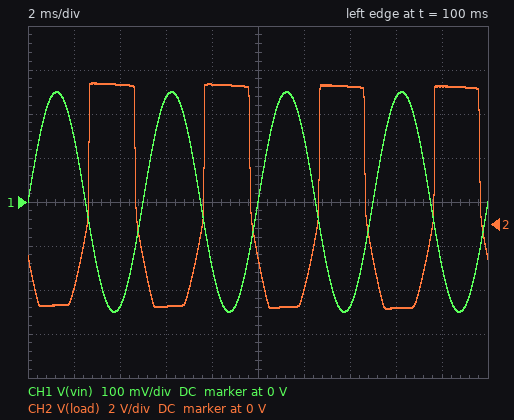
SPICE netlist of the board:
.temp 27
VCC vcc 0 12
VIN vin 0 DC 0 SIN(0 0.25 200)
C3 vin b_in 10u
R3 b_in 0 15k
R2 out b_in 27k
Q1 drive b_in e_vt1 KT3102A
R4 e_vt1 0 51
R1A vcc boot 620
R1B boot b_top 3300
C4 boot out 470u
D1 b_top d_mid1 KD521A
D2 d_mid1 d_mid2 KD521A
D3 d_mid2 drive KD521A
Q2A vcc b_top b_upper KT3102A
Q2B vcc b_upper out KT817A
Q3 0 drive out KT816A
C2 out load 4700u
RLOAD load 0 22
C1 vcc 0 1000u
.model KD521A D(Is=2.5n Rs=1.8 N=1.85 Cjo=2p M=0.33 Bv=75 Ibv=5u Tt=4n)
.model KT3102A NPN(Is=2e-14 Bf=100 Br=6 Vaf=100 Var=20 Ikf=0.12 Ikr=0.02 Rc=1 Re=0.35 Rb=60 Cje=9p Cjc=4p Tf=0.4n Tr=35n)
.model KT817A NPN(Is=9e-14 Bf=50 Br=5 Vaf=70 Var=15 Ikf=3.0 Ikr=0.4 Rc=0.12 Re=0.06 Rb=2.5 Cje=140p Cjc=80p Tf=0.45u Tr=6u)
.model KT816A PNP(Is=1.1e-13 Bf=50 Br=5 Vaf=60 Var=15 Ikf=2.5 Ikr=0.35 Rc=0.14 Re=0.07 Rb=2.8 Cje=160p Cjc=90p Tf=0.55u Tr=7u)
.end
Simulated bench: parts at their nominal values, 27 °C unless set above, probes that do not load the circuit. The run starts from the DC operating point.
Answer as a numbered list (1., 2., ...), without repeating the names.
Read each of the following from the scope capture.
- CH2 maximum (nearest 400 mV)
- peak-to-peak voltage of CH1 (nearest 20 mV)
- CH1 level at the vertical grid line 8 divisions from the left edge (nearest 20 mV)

1. 6.4 V
2. 500 mV
3. 240 mV
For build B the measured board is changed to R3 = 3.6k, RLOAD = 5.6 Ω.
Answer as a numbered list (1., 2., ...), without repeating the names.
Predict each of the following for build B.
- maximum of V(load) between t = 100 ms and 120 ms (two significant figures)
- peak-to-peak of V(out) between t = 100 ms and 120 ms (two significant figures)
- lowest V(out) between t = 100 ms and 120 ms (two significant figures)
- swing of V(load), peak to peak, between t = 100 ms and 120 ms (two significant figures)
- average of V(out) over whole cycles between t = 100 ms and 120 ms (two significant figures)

1. 3.0 V
2. 4.7 V
3. 6.4 V
4. 4.8 V
5. 8.2 V
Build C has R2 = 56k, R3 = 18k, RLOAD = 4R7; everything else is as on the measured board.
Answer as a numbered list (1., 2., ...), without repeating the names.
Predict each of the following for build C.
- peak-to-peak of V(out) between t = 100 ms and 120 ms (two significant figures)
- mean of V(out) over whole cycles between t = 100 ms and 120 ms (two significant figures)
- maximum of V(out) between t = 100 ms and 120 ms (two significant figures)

1. 5.9 V
2. 6.6 V
3. 11 V
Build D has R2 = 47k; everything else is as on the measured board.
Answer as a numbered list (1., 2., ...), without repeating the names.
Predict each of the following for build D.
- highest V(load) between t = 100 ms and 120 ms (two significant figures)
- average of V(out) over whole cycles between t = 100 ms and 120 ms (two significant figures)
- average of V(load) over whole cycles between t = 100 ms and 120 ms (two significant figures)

1. 5.8 V
2. 6.1 V
3. 640 mV
